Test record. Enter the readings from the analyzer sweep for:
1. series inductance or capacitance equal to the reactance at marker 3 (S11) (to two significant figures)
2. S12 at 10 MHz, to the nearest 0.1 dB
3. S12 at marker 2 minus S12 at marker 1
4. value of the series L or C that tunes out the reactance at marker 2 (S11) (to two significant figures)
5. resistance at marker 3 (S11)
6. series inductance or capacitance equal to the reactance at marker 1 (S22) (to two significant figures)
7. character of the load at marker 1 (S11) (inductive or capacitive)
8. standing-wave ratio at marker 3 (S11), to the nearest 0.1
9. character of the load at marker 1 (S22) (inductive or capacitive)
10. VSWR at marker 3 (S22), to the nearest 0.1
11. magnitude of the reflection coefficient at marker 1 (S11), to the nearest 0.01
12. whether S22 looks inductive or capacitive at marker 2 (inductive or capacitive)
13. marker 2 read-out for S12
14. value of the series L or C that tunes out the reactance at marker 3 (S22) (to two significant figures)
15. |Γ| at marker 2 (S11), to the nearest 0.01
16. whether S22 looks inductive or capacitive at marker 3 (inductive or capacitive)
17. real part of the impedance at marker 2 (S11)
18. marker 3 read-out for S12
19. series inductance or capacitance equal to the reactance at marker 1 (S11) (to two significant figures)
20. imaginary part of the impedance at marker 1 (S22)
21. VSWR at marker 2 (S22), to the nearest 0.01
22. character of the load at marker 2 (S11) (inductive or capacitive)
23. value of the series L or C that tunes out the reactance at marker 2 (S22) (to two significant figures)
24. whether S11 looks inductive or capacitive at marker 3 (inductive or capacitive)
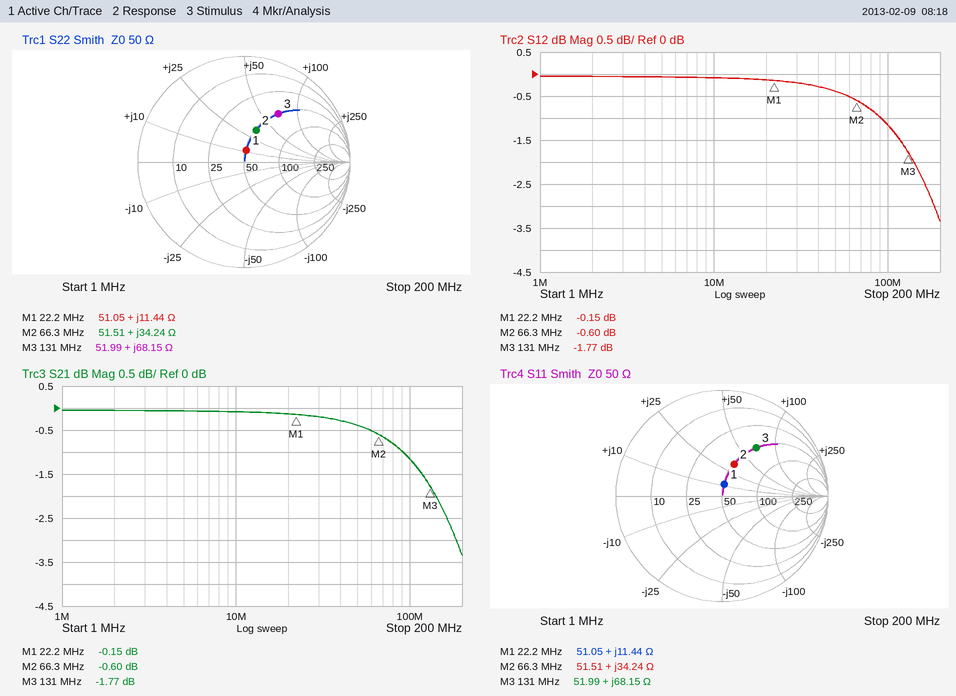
83 nH
-0.1 dB
-0.45 dB
70 pF
51.99 Ω
82 nH
inductive
3.5
inductive
3.5
0.11
inductive
-0.60 dB
18 pF
0.32
inductive
51.51 Ω
-1.77 dB
82 nH
+11.44 Ω
1.94
inductive
70 pF
inductive
